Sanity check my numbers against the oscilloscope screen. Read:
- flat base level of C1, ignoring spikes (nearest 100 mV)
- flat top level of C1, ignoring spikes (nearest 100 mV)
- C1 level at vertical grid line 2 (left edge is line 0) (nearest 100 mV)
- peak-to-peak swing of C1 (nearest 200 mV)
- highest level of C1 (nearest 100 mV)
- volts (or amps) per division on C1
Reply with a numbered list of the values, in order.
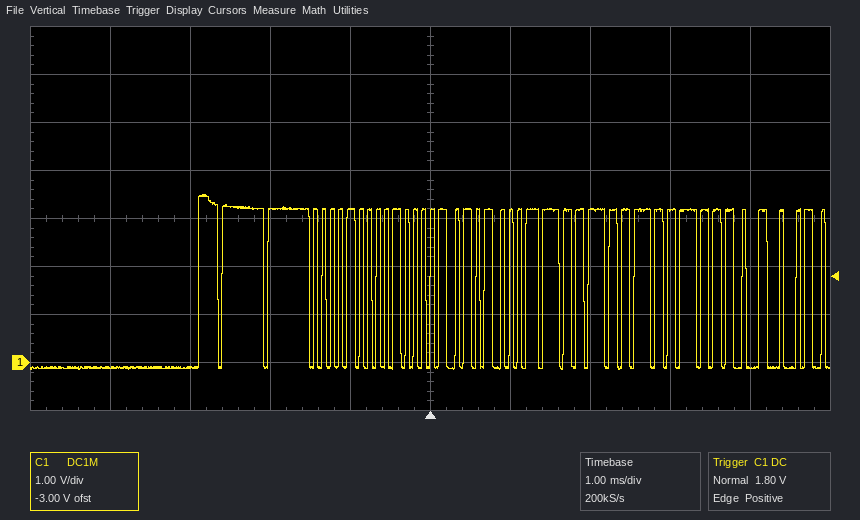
1. -100 mV
2. 3.2 V
3. -100 mV
4. 3.6 V
5. 3.5 V
6. 1 V
